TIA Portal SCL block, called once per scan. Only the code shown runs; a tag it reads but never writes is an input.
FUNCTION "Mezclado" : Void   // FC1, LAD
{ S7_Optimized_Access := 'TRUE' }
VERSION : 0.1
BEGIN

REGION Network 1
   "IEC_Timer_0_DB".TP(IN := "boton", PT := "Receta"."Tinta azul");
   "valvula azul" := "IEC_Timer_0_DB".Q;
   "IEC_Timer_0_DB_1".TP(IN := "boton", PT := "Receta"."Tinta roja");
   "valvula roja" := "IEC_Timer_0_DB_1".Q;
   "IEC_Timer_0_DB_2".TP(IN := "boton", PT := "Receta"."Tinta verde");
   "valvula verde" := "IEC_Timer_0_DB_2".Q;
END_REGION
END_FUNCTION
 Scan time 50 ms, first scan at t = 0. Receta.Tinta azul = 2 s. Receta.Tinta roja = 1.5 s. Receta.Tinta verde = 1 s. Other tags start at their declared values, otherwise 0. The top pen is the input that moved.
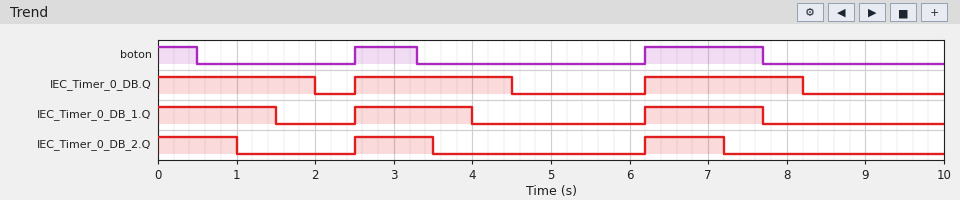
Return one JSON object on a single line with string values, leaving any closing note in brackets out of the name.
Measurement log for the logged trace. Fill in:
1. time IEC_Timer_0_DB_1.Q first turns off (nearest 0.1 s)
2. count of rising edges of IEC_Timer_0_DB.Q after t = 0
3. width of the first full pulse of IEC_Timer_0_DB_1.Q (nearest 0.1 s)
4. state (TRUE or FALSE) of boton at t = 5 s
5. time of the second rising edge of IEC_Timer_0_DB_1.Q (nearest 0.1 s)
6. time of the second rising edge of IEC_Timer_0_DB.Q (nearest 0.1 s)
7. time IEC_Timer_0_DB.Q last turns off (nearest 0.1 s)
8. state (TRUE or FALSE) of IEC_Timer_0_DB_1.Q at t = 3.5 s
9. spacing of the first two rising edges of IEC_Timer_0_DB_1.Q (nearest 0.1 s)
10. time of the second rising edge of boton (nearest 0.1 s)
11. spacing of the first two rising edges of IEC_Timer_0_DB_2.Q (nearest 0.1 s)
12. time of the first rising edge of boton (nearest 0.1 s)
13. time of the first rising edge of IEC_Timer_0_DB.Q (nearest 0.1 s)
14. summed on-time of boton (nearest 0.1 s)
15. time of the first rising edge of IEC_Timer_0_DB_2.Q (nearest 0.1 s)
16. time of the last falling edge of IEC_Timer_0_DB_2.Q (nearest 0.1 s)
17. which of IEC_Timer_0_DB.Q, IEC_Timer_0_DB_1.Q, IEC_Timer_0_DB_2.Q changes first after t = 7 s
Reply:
{"time IEC_Timer_0_DB_1.Q first turns off": "1.5 s", "count of rising edges of IEC_Timer_0_DB.Q after t = 0": "2", "width of the first full pulse of IEC_Timer_0_DB_1.Q": "1.5 s", "state (TRUE or FALSE) of boton at t = 5 s": "FALSE", "time of the second rising edge of IEC_Timer_0_DB_1.Q": "6.2 s", "time of the second rising edge of IEC_Timer_0_DB.Q": "6.2 s", "time IEC_Timer_0_DB.Q last turns off": "8.2 s", "state (TRUE or FALSE) of IEC_Timer_0_DB_1.Q at t = 3.5 s": "TRUE", "spacing of the first two rising edges of IEC_Timer_0_DB_1.Q": "3.7 s", "time of the second rising edge of boton": "6.2 s", "spacing of the first two rising edges of IEC_Timer_0_DB_2.Q": "3.7 s", "time of the first rising edge of boton": "2.5 s", "time of the first rising edge of IEC_Timer_0_DB.Q": "2.5 s", "summed on-time of boton": "2.8 s", "time of the first rising edge of IEC_Timer_0_DB_2.Q": "2.5 s", "time of the last falling edge of IEC_Timer_0_DB_2.Q": "7.2 s", "which of IEC_Timer_0_DB.Q, IEC_Timer_0_DB_1.Q, IEC_Timer_0_DB_2.Q changes first after t = 7 s": "IEC_Timer_0_DB_2.Q"}
